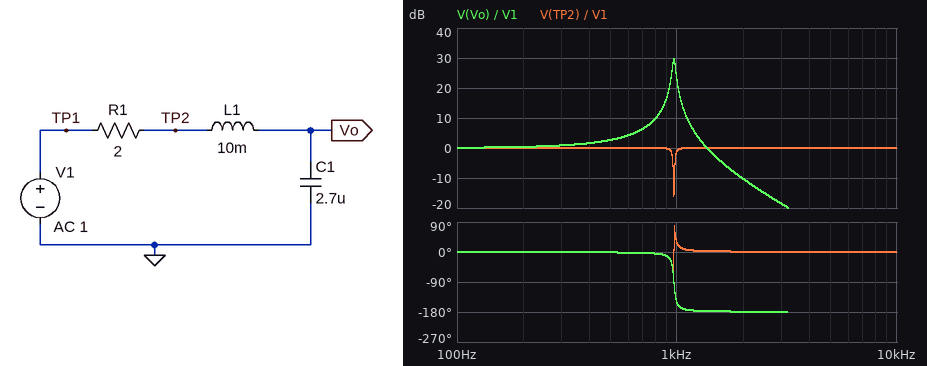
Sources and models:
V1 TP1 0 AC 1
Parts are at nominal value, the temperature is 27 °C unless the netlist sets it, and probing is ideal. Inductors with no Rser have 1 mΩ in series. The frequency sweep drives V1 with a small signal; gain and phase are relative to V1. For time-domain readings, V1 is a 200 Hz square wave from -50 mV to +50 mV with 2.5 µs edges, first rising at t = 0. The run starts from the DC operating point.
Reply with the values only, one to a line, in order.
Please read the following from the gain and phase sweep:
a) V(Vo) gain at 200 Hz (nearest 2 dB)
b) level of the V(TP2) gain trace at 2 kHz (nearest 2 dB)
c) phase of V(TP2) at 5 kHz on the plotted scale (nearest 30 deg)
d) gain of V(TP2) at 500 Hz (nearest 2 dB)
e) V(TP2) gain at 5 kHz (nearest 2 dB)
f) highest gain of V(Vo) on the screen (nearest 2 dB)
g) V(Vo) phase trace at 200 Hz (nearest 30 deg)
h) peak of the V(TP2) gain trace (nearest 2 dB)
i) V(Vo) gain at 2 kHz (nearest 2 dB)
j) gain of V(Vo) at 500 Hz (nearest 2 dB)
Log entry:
0 dB
0 dB
0 deg
0 dB
0 dB
30 dB
0 deg
0 dB
-10 dB
2 dB
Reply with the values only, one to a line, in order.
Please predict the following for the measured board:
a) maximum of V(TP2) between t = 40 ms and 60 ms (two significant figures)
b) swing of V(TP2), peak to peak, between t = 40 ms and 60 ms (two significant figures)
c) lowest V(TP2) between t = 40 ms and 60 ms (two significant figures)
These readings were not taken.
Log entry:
56 mV
110 mV
-56 mV
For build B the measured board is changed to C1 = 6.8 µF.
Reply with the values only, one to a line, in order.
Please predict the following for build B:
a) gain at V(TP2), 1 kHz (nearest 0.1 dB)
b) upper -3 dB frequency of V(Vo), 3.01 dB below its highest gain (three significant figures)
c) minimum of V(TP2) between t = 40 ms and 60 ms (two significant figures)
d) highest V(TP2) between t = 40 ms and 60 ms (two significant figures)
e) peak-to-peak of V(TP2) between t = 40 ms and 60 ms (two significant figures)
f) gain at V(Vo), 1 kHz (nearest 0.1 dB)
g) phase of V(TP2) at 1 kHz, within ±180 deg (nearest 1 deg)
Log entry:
0 dB
626 Hz
-68 mV
68 mV
140 mV
-4.5 dB
3 deg
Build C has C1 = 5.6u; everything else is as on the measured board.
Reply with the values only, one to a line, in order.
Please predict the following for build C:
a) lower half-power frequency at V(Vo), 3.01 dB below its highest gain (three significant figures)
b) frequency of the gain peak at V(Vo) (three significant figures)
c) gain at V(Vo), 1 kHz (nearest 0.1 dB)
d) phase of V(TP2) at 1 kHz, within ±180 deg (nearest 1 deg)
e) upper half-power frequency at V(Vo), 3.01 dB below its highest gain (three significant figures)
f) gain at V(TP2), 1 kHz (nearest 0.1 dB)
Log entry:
656 Hz
672 Hz
-1.7 dB
3 deg
688 Hz
0 dB
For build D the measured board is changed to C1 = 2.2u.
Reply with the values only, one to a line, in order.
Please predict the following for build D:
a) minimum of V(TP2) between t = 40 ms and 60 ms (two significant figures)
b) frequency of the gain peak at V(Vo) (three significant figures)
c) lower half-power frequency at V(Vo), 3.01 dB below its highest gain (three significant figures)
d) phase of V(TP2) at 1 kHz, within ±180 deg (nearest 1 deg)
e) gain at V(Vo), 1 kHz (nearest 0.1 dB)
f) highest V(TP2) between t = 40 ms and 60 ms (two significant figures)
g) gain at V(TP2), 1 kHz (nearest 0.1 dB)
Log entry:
-53 mV
1.07 kHz
1.06 kHz
-12 deg
17.4 dB
53 mV
-0.2 dB
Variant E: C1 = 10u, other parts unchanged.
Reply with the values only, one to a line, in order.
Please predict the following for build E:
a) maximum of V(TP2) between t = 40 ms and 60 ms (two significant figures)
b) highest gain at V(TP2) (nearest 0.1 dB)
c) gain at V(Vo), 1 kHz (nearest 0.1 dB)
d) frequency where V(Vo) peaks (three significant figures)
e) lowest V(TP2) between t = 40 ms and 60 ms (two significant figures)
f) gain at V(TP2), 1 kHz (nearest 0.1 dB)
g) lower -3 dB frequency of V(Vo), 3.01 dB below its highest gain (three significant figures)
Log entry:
54 mV
0 dB
-9.4 dB
503 Hz
-54 mV
0 dB
487 Hz
